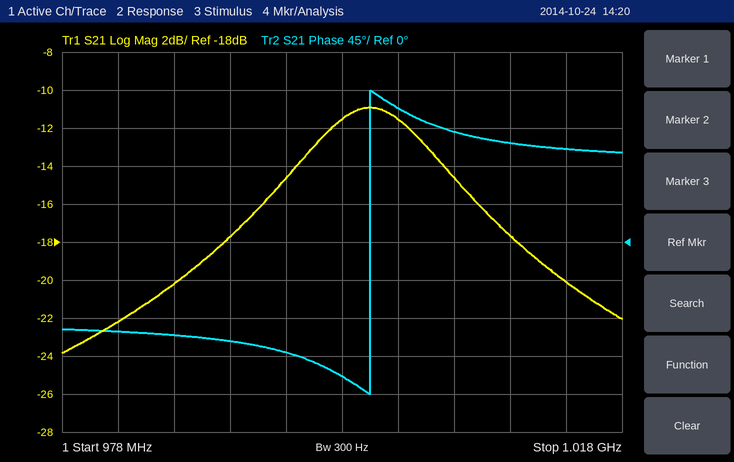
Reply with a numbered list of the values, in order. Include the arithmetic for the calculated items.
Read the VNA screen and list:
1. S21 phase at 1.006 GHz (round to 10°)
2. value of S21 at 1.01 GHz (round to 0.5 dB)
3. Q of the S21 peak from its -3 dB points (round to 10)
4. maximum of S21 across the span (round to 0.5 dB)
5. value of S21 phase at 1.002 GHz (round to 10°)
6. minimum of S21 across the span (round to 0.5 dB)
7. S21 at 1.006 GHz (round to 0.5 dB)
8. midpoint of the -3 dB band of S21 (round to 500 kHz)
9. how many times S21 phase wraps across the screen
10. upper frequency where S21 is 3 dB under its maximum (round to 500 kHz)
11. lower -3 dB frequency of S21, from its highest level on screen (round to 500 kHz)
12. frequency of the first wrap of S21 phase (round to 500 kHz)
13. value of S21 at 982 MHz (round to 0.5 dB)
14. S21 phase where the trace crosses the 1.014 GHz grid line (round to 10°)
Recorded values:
1. 130°
2. -17.5 dB
3. 1 GHz / 10 MHz ≈ 100
4. -11.0 dB
5. 160°
6. -24.0 dB
7. -14.5 dB
8. 1.0000 GHz
9. 1
10. 1.0050 GHz
11. 995.0 MHz
12. 1.0000 GHz
13. -22.0 dB
14. 110°
